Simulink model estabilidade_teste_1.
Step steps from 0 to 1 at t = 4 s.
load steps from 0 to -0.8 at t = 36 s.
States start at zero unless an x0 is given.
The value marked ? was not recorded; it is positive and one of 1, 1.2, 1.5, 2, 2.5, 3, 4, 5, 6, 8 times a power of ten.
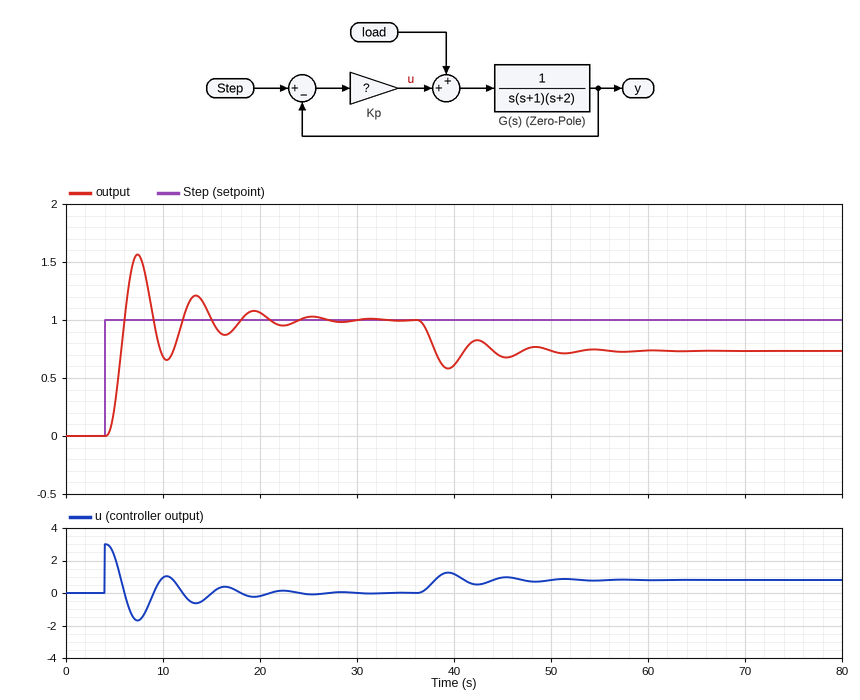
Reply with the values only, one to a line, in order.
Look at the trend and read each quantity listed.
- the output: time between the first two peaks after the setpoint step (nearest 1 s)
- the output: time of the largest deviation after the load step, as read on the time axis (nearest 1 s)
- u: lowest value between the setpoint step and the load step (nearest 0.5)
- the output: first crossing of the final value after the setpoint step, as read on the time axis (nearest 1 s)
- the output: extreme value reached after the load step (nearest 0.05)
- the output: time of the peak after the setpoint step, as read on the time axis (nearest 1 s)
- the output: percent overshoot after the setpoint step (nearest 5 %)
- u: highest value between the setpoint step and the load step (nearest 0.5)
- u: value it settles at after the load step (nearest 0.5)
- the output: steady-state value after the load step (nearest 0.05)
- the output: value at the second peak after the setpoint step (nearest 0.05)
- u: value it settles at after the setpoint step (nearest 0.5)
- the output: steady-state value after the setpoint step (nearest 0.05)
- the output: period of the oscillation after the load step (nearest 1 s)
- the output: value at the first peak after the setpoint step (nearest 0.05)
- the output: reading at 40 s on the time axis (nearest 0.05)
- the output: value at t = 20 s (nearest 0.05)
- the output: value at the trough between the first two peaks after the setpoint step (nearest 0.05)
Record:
6 s
39 s
-1.5
6 s
0.60
7 s
55 %
3.0
1.0
0.75
1.20
0.0
1.00
6 s
1.55
0.60
1.05
0.65
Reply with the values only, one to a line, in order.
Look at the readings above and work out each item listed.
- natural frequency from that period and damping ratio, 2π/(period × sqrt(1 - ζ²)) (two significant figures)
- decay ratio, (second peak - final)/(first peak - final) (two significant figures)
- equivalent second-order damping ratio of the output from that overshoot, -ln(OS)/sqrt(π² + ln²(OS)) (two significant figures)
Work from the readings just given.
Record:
1.1 rad/s
0.36
0.19
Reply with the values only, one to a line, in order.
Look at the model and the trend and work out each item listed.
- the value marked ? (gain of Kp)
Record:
3
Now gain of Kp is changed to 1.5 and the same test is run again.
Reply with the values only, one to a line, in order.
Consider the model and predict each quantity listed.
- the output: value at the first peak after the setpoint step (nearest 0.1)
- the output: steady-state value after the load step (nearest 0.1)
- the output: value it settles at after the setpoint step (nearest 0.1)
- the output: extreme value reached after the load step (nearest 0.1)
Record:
1.3
0.5
1.0
0.3
